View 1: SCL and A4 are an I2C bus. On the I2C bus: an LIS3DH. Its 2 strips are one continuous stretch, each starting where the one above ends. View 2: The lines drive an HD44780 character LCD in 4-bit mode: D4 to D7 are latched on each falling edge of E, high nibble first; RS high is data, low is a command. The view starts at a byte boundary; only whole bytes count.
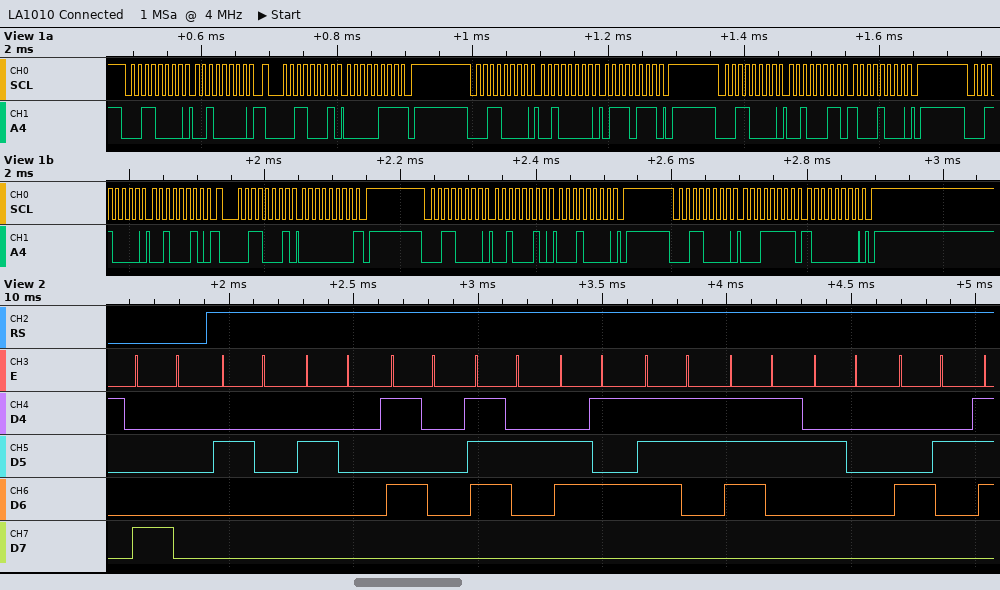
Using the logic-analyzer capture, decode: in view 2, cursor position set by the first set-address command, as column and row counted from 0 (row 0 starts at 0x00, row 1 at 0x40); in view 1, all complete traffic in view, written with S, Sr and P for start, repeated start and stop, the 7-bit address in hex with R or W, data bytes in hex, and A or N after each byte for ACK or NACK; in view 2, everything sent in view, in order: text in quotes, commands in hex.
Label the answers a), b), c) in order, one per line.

a) column 0, row 0
b) S 18W A 20 A Sr 18R A 07 N P S 18W A 20 A 77 A P S 18W A 23 A 88 A P S 18W A 22 A Sr 18R A 00 N P S 18W A 22 A 10 A P S 18W A 1F A 80 A P
c) 0x80 "  Press B"
